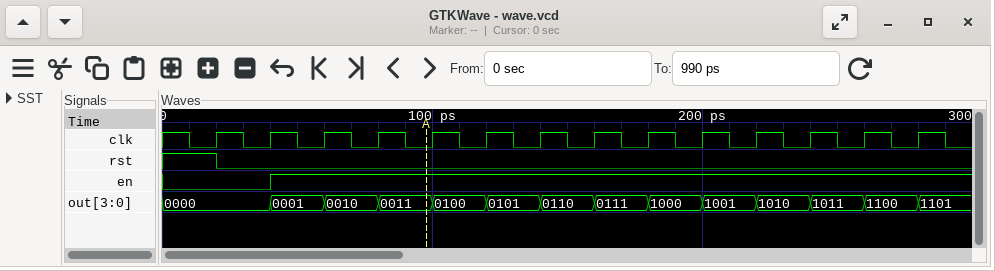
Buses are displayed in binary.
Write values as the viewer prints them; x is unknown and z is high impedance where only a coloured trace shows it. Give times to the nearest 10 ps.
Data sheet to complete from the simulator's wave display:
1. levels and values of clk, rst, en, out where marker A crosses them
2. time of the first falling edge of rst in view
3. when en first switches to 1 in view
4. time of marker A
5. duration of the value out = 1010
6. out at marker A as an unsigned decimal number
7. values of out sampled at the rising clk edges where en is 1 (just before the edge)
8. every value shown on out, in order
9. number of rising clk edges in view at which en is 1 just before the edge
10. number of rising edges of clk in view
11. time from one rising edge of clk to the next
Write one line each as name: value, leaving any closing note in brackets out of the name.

levels and values of clk, rst, en, out where marker A crosses them: clk=0, rst=0, en=1, out=0011
time of the first falling edge of rst in view: 20 ps
when en first switches to 1 in view: 40 ps
time of marker A: 100 ps
duration of the value out = 1010: 20 ps
out at marker A as an unsigned decimal number: 3
values of out sampled at the rising clk edges where en is 1: 0001, 0010, 0011, 0100, 0101, 0110, 0111, 1000, 1001, 1010, 1011, 1100
every value shown on out, in order: 0000, 0001, 0010, 0011, 0100, 0101, 0110, 0111, 1000, 1001, 1010, 1011, 1100, 1101
number of rising clk edges in view at which en is 1 just before the edge: 12
number of rising edges of clk in view: 14
time from one rising edge of clk to the next: 20 ps
